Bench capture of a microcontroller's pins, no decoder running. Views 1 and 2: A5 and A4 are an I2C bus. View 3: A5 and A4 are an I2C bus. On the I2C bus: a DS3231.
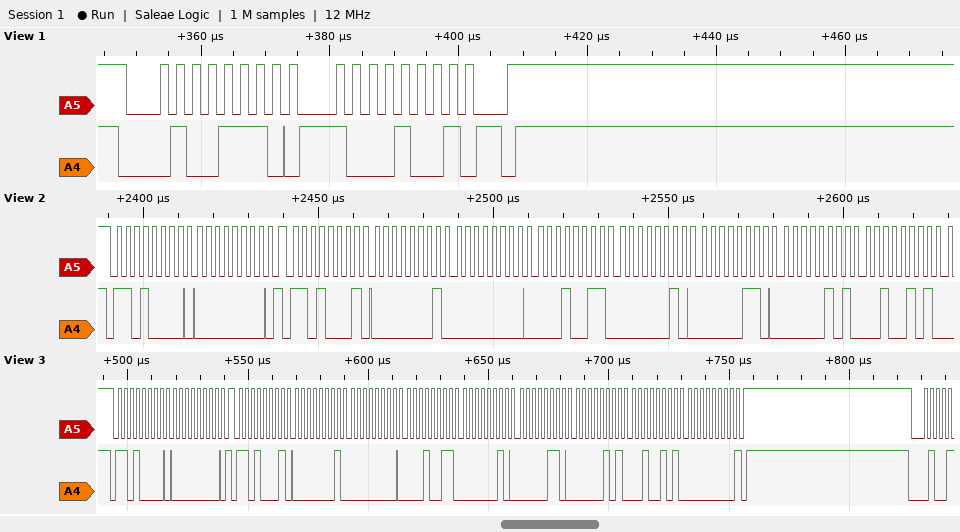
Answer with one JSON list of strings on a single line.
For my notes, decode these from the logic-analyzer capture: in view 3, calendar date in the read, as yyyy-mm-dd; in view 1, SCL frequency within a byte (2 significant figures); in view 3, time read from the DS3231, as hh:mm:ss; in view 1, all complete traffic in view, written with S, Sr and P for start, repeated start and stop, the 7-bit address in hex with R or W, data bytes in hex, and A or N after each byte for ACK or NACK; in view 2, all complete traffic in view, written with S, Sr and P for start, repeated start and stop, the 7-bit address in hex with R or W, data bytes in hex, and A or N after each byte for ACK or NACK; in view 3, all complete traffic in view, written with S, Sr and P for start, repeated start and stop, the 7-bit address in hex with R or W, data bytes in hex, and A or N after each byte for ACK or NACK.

["2025-05-06", "400 kHz", "13:00:01", "S 27W A 89 A P", "S 68W A 00 A Sr 68R A 01 A 00 A 13 A 02 A 06 A 05 A 25 A", "S 68W A 00 A Sr 68R A 01 A 00 A 13 A 02 A 06 A 05 A 25 A 00 N P"]
